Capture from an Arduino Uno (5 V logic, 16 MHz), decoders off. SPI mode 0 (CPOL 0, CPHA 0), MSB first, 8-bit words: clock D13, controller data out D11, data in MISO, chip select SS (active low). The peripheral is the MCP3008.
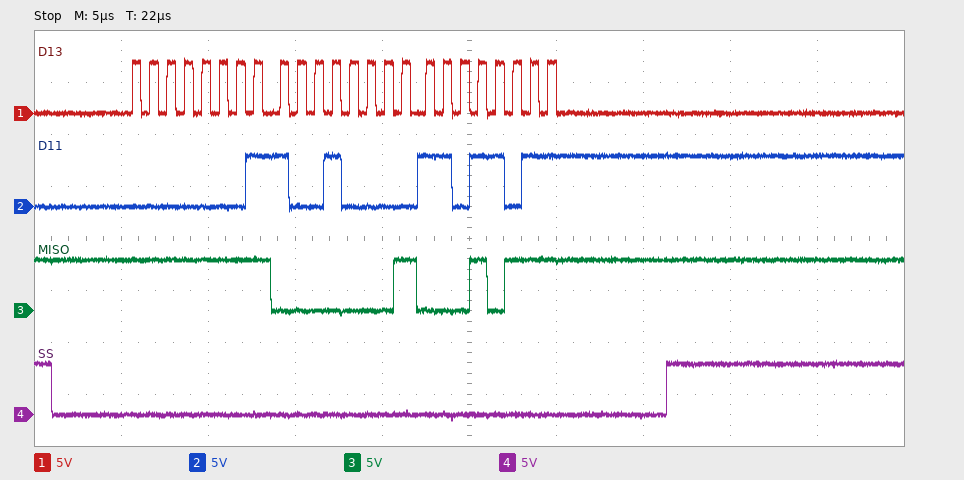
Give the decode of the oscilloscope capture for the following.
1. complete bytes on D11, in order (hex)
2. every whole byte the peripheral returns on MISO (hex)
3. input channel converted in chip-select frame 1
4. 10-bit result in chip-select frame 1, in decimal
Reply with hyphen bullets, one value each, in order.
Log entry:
- 01 90 DB
- FF 01 17
- 1
- 279
